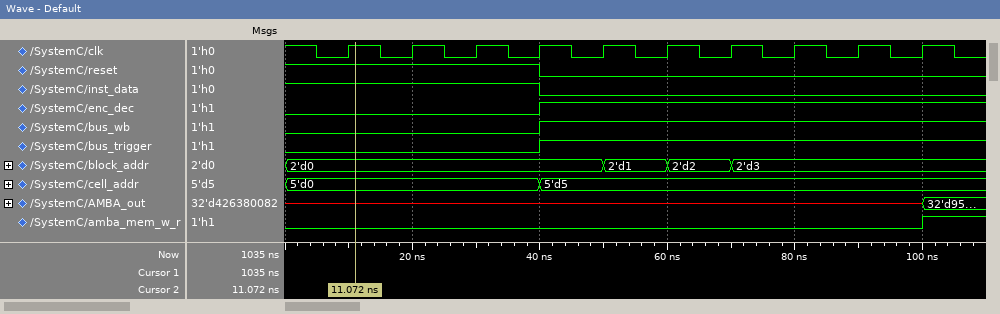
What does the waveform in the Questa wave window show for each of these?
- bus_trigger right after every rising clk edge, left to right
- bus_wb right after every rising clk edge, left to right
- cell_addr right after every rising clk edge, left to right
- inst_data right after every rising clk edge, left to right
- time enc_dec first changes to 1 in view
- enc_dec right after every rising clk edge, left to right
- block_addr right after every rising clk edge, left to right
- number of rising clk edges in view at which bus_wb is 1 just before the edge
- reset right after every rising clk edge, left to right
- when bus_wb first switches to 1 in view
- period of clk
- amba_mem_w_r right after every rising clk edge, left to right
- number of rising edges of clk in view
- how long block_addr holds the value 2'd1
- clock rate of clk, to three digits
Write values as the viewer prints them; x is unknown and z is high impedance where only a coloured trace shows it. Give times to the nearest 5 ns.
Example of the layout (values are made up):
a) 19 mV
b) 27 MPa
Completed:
a) 0 0 0 1 1 1 1 1 1 1
b) 0 0 0 1 1 1 1 1 1 1
c) 5'd0, 5'd0, 5'd0, 5'd5, 5'd5, 5'd5, 5'd5, 5'd5, 5'd5, 5'd5
d) 1 1 1 0 0 0 0 0 0 0
e) 40 ns
f) 0 0 0 1 1 1 1 1 1 1
g) 2'd0, 2'd0, 2'd0, 2'd0, 2'd1, 2'd2, 2'd3, 2'd3, 2'd3, 2'd3
h) 6
i) 1 1 1 0 0 0 0 0 0 0
j) 40 ns
k) 10 ns
l) 0 0 0 0 0 0 0 0 0 1
m) 10
n) 10 ns
o) 100 MHz
